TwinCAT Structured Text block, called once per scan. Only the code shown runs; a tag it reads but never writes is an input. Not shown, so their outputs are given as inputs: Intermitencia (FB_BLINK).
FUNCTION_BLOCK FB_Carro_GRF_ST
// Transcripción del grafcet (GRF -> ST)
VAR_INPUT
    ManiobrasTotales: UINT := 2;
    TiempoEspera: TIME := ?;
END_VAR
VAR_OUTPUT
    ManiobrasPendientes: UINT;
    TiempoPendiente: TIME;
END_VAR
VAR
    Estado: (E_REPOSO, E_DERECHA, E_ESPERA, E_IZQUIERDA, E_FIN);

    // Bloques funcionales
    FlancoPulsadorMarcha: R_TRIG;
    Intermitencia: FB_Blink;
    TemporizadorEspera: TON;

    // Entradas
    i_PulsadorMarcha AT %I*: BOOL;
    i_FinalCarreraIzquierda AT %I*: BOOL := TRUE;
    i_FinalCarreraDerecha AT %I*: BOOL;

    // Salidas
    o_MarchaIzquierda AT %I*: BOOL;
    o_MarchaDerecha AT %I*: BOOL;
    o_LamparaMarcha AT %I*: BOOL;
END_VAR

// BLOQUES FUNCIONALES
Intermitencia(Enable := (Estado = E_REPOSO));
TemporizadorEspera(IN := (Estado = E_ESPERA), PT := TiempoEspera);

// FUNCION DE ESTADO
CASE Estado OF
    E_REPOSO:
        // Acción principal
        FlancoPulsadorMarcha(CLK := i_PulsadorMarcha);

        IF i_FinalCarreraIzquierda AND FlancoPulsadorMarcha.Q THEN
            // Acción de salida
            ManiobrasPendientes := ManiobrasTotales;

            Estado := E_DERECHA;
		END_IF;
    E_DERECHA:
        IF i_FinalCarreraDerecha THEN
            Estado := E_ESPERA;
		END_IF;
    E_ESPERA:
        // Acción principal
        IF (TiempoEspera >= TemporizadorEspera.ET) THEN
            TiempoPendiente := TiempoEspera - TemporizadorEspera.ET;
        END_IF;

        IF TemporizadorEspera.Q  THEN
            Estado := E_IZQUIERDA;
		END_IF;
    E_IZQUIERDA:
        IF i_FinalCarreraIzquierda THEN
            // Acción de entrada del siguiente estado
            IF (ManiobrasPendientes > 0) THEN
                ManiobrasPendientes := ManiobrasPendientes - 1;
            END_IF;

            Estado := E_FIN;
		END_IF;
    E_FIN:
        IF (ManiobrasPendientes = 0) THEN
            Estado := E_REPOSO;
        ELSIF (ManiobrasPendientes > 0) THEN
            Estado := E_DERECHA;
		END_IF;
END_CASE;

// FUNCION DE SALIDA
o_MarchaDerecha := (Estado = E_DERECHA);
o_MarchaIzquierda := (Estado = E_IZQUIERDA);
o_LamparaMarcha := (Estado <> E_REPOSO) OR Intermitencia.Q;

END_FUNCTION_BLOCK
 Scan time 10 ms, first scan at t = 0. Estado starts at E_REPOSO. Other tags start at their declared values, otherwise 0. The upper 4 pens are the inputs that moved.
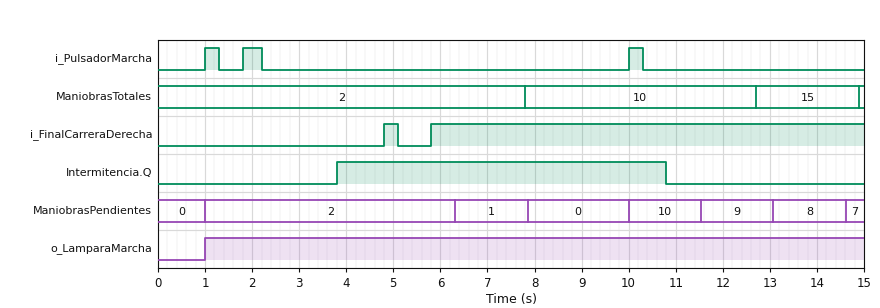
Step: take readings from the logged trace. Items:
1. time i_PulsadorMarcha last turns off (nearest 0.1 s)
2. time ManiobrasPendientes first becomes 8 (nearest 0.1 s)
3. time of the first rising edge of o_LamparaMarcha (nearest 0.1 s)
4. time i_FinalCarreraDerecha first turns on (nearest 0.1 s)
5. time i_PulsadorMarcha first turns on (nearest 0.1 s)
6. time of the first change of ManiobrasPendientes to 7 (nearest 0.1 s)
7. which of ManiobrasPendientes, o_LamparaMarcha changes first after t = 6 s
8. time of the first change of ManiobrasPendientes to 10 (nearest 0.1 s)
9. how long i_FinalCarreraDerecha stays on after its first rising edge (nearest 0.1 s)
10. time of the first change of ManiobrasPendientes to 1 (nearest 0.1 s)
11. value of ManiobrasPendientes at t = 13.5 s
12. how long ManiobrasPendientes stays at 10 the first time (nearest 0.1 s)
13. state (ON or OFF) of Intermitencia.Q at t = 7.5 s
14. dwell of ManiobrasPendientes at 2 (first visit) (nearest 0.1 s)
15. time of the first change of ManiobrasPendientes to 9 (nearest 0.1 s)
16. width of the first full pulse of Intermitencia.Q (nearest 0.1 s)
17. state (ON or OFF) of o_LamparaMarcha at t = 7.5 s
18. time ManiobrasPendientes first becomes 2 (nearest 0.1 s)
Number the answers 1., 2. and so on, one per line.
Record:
1. 10.3 s
2. 13.1 s
3. 1.0 s
4. 4.8 s
5. 1.0 s
6. 14.6 s
7. ManiobrasPendientes
8. 10.0 s
9. 0.3 s
10. 6.3 s
11. 8
12. 1.5 s
13. ON
14. 5.3 s
15. 11.5 s
16. 7.0 s
17. ON
18. 1.0 s
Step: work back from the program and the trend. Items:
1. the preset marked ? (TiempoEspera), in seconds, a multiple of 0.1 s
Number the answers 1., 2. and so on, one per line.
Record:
1. 1.5 s
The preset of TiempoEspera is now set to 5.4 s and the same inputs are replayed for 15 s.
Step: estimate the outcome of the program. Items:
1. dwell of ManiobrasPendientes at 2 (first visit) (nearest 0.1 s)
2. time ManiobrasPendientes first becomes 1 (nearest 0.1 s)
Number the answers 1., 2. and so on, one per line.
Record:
1. 9.2 s
2. 10.2 s
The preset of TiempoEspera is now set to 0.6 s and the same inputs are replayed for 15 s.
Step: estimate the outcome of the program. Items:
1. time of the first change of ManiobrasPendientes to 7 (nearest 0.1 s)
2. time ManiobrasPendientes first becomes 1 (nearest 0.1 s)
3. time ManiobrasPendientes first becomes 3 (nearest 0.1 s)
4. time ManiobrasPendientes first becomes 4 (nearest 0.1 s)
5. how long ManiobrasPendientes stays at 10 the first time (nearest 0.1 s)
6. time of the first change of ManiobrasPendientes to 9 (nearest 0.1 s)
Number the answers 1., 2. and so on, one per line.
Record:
1. 11.9 s
2. 5.4 s
3. 14.5 s
4. 13.8 s
5. 0.6 s
6. 10.6 s
